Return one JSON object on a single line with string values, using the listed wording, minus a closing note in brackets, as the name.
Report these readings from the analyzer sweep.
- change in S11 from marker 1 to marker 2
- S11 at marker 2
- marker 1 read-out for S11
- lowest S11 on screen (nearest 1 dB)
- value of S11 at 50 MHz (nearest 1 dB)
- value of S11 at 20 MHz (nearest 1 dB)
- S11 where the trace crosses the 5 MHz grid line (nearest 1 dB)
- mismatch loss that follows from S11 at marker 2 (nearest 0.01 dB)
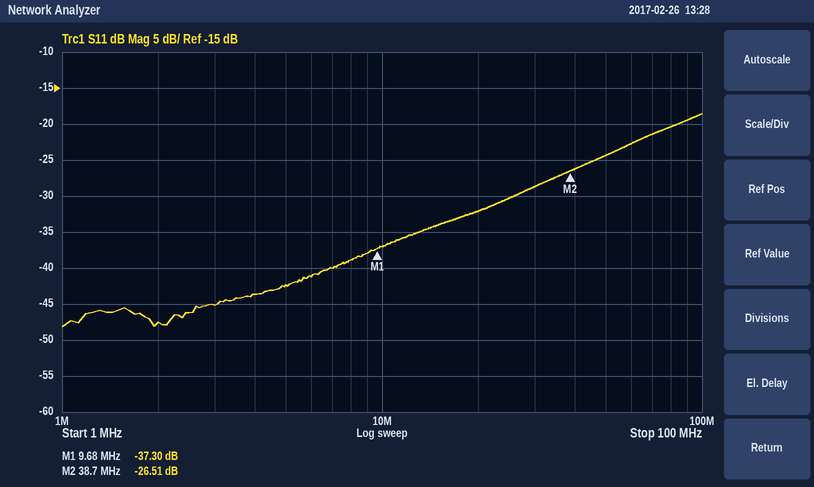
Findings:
{"change in S11 from marker 1 to marker 2": "10.79 dB", "S11 at marker 2": "-26.51 dB", "marker 1 read-out for S11": "-37.30 dB", "lowest S11 on screen": "-48 dB", "value of S11 at 50 MHz": "-24 dB", "value of S11 at 20 MHz": "-32 dB", "S11 where the trace crosses the 5 MHz grid line": "-42 dB", "mismatch loss that follows from S11 at marker 2": "0.01 dB"}
